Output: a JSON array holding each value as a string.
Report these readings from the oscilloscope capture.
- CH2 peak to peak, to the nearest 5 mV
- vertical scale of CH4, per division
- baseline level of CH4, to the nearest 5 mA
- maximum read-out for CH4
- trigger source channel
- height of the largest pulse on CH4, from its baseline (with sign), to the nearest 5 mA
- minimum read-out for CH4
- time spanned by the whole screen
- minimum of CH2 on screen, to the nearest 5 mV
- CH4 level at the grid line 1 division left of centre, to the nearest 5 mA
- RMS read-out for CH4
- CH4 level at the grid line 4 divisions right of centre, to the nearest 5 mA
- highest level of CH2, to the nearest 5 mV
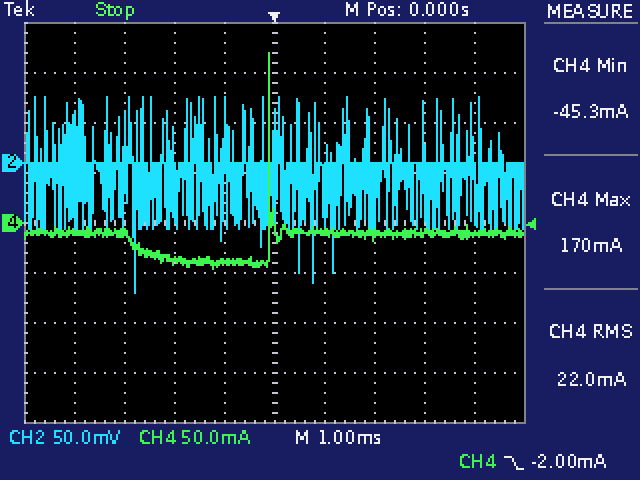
["195 mV", "50 mA", "-10 mA", "170 mA", "CH4", "+180 mA", "-45.3 mA", "10 ms", "-130 mV", "-40 mA", "22.0 mA", "-10 mA", "65 mV"]
